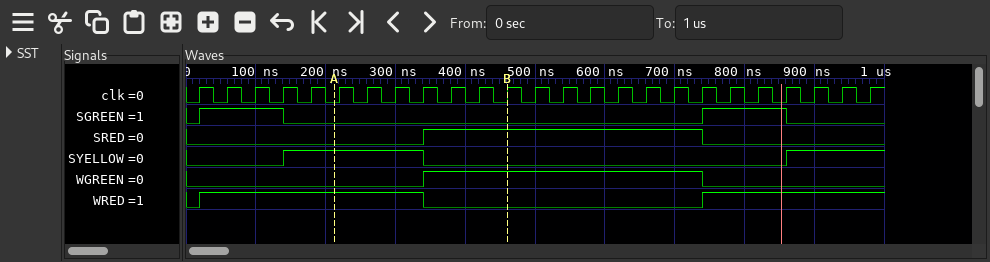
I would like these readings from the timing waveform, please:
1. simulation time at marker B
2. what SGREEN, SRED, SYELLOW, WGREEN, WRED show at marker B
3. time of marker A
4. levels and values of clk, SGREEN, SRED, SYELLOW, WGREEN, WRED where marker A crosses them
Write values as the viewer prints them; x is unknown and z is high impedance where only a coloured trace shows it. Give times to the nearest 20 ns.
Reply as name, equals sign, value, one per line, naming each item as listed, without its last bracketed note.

simulation time at marker B = 460 ns
what SGREEN, SRED, SYELLOW, WGREEN, WRED show at marker B = SGREEN=0, SRED=1, SYELLOW=0, WGREEN=1, WRED=0
time of marker A = 220 ns
levels and values of clk, SGREEN, SRED, SYELLOW, WGREEN, WRED where marker A crosses them = clk=0, SGREEN=0, SRED=0, SYELLOW=1, WGREEN=0, WRED=1
